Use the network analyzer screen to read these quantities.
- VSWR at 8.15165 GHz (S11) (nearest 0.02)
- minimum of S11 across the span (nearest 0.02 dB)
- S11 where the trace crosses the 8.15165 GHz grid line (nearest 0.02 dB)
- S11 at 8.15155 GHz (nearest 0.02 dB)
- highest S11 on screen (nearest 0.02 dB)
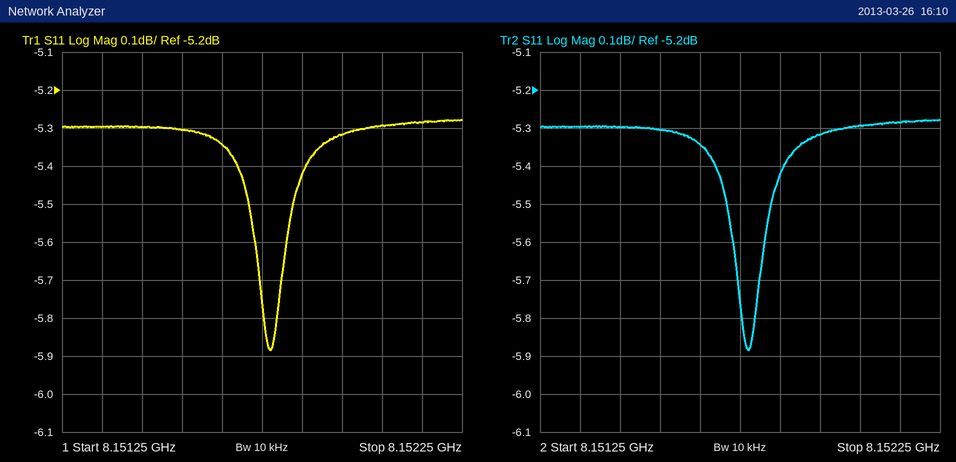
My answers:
3.36
-5.88 dB
-5.34 dB
-5.30 dB
-5.28 dB
